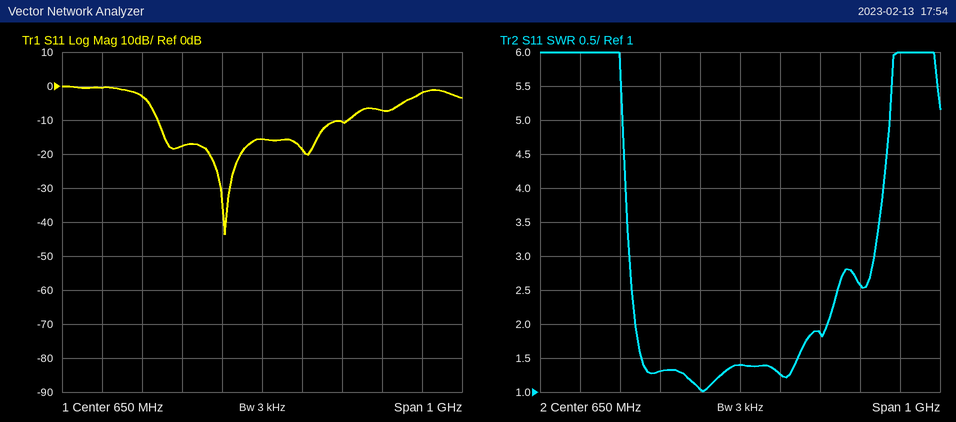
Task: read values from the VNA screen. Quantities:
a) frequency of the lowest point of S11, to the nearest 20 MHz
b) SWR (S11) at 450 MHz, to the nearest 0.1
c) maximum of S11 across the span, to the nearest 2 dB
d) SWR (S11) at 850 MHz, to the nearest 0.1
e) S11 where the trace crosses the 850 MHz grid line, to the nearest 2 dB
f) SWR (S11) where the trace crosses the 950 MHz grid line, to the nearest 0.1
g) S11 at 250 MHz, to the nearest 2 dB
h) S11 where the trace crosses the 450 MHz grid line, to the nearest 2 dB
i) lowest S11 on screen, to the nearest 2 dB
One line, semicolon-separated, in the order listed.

560 MHz; 1.3; 0 dB; 1.9; -10 dB; 2.6; 0 dB; -18 dB; -44 dB
